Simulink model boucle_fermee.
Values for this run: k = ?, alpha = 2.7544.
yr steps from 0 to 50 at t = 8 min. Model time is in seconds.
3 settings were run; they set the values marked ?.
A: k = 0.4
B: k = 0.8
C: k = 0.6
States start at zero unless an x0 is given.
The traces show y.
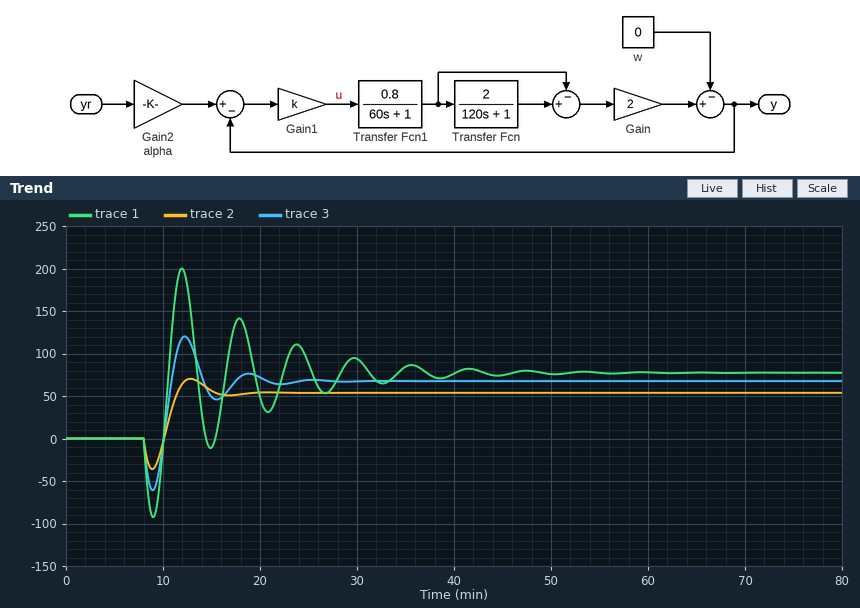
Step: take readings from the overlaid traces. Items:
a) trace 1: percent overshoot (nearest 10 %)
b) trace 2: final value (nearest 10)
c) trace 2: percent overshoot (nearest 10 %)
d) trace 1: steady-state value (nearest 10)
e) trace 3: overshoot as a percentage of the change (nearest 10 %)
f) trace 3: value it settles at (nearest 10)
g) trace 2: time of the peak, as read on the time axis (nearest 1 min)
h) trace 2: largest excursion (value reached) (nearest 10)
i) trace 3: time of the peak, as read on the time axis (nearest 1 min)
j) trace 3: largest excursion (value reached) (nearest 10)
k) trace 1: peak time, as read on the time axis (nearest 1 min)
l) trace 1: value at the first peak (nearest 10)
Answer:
160 %
50
30 %
80
80 %
70
13 min
70
12 min
120
12 min
200
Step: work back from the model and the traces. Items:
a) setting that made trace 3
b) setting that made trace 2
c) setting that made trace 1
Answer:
C
A
B
